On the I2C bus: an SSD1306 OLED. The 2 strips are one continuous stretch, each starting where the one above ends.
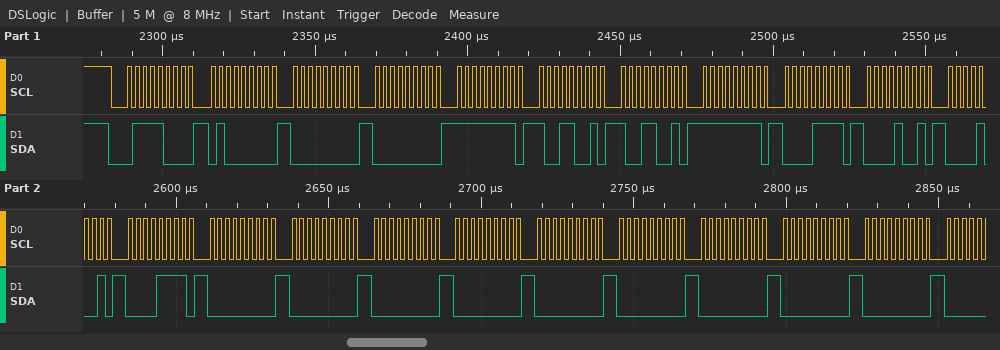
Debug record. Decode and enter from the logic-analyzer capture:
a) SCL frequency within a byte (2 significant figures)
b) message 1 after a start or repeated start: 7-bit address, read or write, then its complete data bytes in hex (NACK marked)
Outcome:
400 kHz
0x3C write: 40 00 00 FF 99 99 FF 0F 09 09 0F 00 00 00 00 00 00 00 00 00
